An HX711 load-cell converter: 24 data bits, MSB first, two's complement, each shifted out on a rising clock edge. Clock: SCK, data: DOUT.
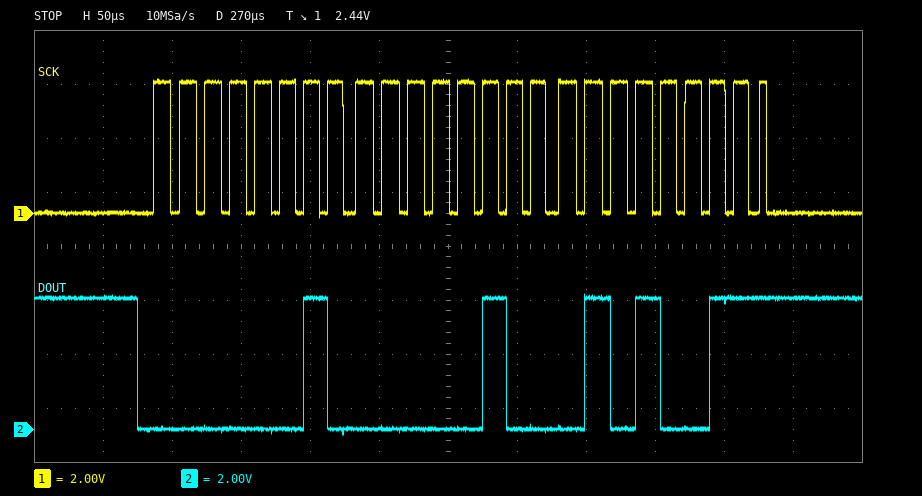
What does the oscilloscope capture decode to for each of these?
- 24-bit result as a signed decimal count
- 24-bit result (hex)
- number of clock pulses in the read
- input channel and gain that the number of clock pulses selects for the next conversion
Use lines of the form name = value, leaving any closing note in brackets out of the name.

24-bit result as a signed decimal count = 132179
24-bit result = 0x020453
number of clock pulses in the read = 25
input channel and gain that the number of clock pulses selects for the next conversion = channel A, gain 128
